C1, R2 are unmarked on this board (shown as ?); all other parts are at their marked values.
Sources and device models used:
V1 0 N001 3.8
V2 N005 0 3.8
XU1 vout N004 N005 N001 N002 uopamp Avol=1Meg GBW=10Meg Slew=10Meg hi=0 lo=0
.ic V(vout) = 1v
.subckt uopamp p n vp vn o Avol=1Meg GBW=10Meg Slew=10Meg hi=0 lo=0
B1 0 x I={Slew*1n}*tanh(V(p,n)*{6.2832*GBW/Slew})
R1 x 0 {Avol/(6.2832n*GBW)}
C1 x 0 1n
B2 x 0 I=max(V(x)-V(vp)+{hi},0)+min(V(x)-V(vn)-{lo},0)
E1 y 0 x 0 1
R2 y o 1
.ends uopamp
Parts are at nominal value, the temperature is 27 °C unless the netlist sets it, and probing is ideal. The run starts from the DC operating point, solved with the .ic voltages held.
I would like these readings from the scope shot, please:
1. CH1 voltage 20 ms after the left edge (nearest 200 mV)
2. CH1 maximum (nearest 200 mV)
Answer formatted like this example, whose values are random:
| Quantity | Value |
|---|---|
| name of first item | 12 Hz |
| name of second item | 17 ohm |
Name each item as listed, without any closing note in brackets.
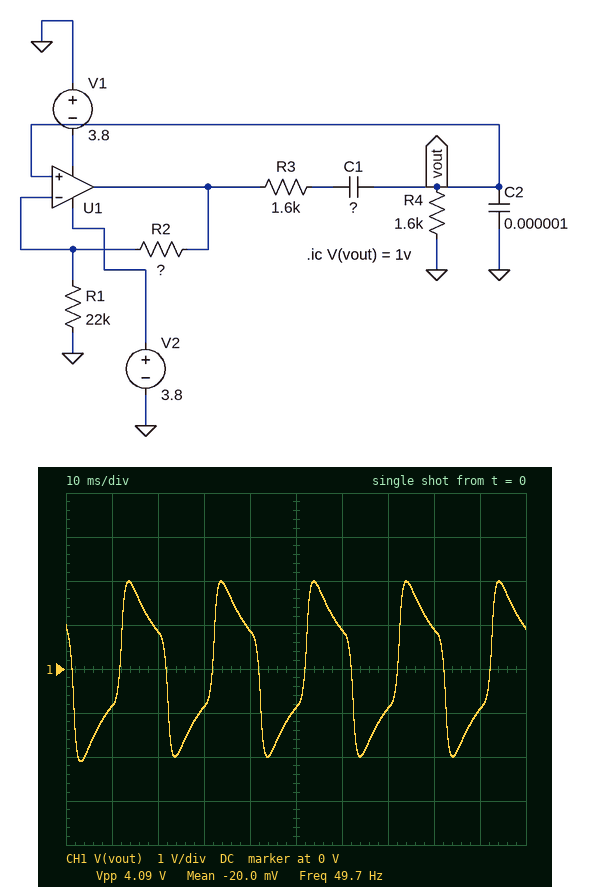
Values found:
| Quantity | Value |
|---|---|
| CH1 voltage 20 ms after the left edge | 800 mV |
| CH1 maximum | 2.0 V |
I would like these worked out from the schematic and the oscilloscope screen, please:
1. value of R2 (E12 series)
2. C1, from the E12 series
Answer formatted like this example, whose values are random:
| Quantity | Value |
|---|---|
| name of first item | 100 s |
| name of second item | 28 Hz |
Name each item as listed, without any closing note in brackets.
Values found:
| Quantity | Value |
|---|---|
| value of R2 | 82 kΩ |
| C1, from the E12 series | 1.8 µF |
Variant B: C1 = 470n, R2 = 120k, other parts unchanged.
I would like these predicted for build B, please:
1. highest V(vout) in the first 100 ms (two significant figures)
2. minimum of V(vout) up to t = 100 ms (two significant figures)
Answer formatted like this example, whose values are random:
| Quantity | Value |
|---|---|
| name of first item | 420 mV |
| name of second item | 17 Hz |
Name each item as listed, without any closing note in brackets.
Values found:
| Quantity | Value |
|---|---|
| highest V(vout) in the first 100 ms | 1.2 V |
| minimum of V(vout) up to t = 100 ms | -1.2 V |
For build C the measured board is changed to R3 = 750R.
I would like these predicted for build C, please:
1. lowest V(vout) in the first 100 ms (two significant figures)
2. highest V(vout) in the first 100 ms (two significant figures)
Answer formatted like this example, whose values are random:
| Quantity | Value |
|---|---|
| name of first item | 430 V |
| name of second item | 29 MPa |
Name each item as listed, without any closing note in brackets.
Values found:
| Quantity | Value |
|---|---|
| lowest V(vout) in the first 100 ms | -2.7 V |
| highest V(vout) in the first 100 ms | 2.7 V |
